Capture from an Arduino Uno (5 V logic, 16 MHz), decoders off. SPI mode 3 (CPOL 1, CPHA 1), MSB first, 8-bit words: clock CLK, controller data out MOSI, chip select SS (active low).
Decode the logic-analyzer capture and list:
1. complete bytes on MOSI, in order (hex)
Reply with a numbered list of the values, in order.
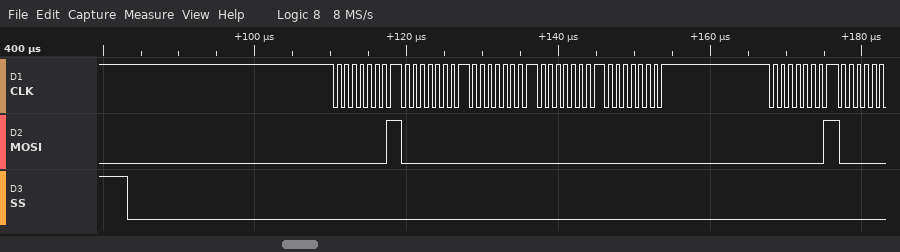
1. 01 00 00 00 00 01
